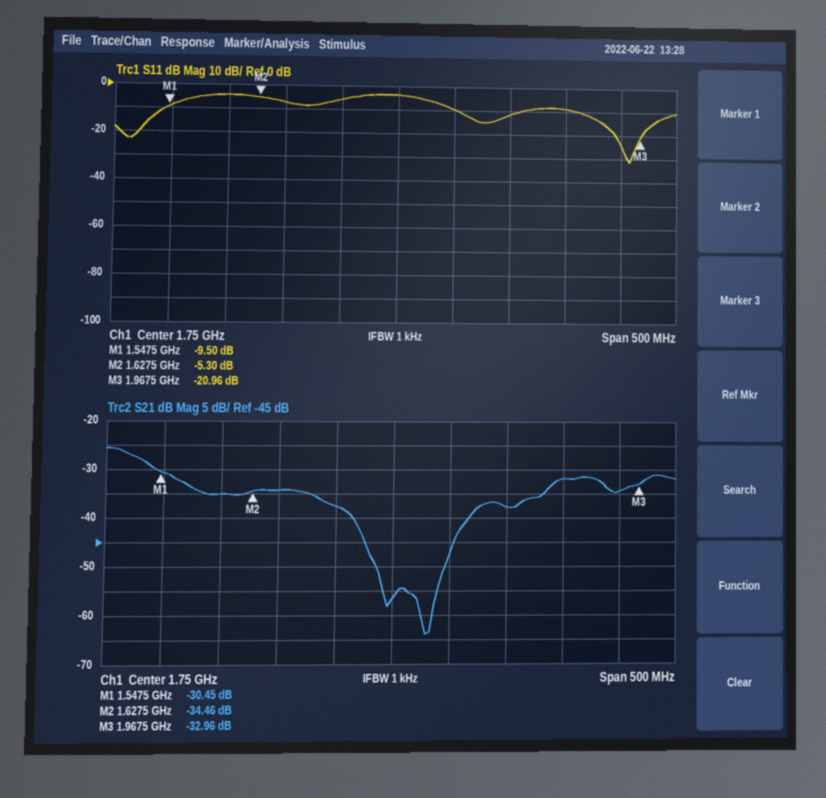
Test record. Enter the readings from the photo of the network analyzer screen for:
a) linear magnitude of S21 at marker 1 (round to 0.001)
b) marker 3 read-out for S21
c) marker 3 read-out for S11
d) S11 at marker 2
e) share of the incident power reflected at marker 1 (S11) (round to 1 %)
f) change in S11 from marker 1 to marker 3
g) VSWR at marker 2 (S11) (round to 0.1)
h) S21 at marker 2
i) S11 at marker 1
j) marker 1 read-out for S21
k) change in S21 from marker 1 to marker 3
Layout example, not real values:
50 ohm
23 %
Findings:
0.030
-32.96 dB
-20.96 dB
-5.30 dB
11 %
-11.46 dB
3.4
-34.46 dB
-9.50 dB
-30.45 dB
-2.51 dB
